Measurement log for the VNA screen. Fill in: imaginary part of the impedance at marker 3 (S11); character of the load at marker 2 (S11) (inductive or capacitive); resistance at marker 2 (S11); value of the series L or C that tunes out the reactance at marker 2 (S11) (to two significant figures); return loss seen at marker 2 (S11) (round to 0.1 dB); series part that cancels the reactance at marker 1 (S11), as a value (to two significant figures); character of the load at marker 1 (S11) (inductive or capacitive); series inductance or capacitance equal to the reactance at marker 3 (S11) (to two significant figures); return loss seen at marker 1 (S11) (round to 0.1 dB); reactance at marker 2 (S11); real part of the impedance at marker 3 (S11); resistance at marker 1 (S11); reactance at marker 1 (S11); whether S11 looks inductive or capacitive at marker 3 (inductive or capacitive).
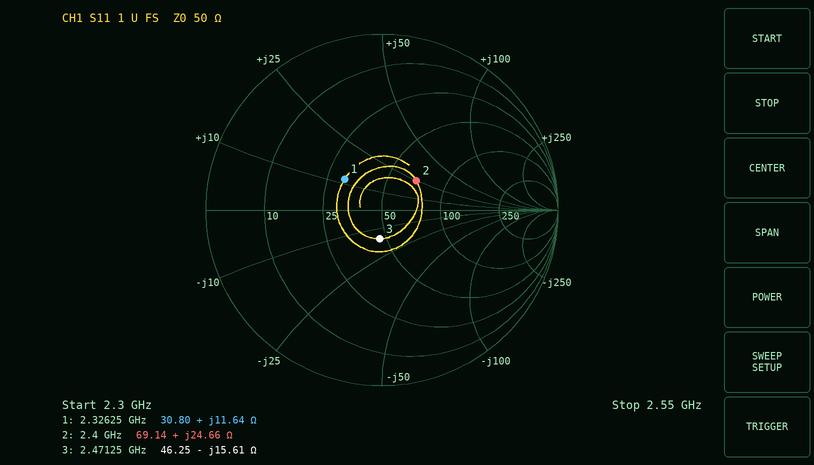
-15.61 Ω
inductive
69.14 Ω
2.7 pF
11.8 dB
5.9 pF
inductive
4.1 pF
11.2 dB
+24.66 Ω
46.25 Ω
30.80 Ω
+11.64 Ω
capacitive
